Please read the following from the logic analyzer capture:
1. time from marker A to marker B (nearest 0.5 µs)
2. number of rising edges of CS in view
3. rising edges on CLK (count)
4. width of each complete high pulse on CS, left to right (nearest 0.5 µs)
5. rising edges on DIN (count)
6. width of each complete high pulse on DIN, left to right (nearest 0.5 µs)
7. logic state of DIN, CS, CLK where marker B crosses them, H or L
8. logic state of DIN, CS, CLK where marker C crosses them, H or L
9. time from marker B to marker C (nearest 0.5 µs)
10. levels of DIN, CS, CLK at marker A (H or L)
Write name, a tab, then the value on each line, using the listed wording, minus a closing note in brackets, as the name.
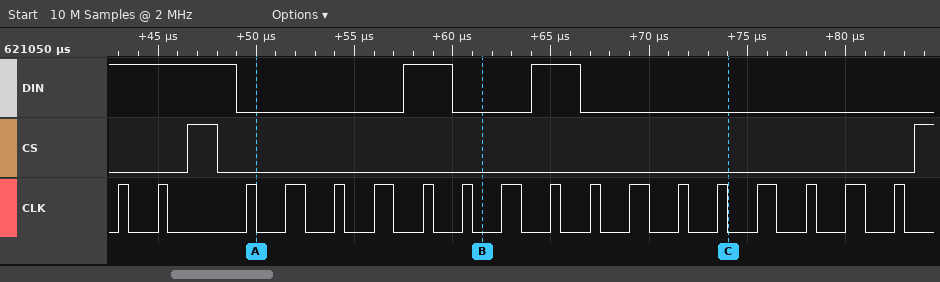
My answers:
time from marker A to marker B	11.5 µs
number of rising edges of CS in view	2
rising edges on CLK	18
width of each complete high pulse on CS, left to right	1.5 µs
rising edges on DIN	2
width of each complete high pulse on DIN, left to right	2.5 µs, 2.5 µs
logic state of DIN, CS, CLK where marker B crosses them, H or L	DIN=L, CS=L, CLK=L
logic state of DIN, CS, CLK where marker C crosses them, H or L	DIN=L, CS=L, CLK=L
time from marker B to marker C	12.5 µs
levels of DIN, CS, CLK at marker A	DIN=L, CS=L, CLK=L
